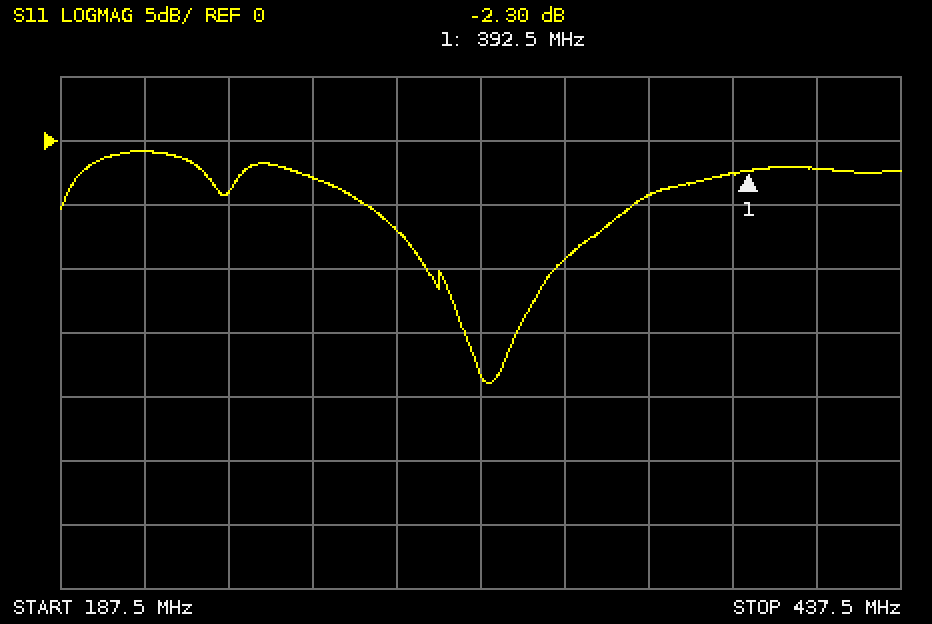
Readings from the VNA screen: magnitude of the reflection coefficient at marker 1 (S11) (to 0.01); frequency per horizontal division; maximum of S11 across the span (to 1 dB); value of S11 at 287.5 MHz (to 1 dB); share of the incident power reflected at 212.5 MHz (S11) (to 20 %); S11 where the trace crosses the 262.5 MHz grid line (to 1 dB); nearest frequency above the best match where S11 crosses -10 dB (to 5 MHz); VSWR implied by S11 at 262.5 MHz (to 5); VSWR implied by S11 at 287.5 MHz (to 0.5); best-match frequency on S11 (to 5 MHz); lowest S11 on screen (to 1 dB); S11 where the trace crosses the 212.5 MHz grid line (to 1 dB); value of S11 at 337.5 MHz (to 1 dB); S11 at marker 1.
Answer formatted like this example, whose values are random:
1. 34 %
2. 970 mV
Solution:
1. 0.77
2. 25 MHz
3. -1 dB
4. -7 dB
5. 80 %
6. -3 dB
7. 335 MHz
8. 5
9. 2.5
10. 315 MHz
11. -19 dB
12. -1 dB
13. -9 dB
14. -2.30 dB
